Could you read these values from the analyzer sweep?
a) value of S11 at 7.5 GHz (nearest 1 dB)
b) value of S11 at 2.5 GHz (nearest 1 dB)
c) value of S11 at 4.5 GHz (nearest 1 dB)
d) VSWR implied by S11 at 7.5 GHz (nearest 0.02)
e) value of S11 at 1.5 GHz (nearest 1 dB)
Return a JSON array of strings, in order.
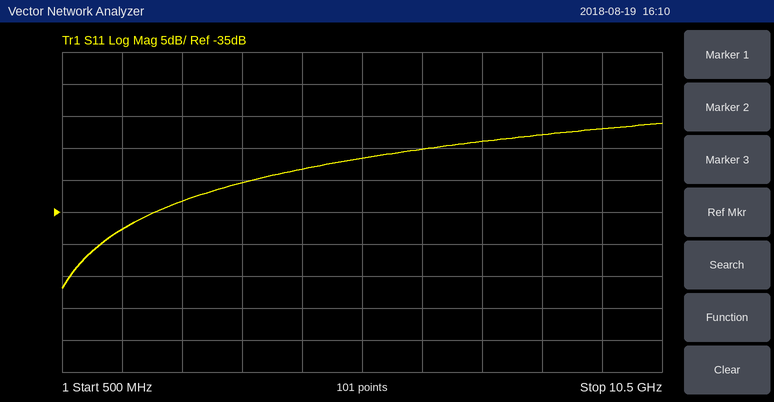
["-24 dB", "-33 dB", "-28 dB", "1.14", "-38 dB"]
